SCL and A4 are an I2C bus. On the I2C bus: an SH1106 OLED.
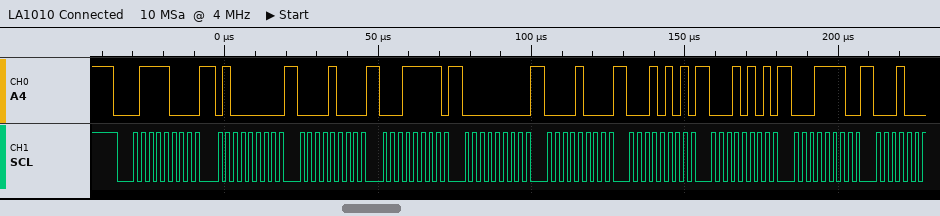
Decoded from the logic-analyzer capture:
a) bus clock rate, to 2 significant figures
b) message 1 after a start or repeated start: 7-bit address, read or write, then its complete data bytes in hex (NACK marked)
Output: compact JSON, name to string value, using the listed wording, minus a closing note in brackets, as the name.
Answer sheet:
{"bus clock rate, to 2 significant figures": "400 kHz", "message 1 after a start or repeated start: 7-bit address, read or write, then its complete data bytes in hex": "0x3C write: 40 08 1F 00 08 15 15 1E"}
